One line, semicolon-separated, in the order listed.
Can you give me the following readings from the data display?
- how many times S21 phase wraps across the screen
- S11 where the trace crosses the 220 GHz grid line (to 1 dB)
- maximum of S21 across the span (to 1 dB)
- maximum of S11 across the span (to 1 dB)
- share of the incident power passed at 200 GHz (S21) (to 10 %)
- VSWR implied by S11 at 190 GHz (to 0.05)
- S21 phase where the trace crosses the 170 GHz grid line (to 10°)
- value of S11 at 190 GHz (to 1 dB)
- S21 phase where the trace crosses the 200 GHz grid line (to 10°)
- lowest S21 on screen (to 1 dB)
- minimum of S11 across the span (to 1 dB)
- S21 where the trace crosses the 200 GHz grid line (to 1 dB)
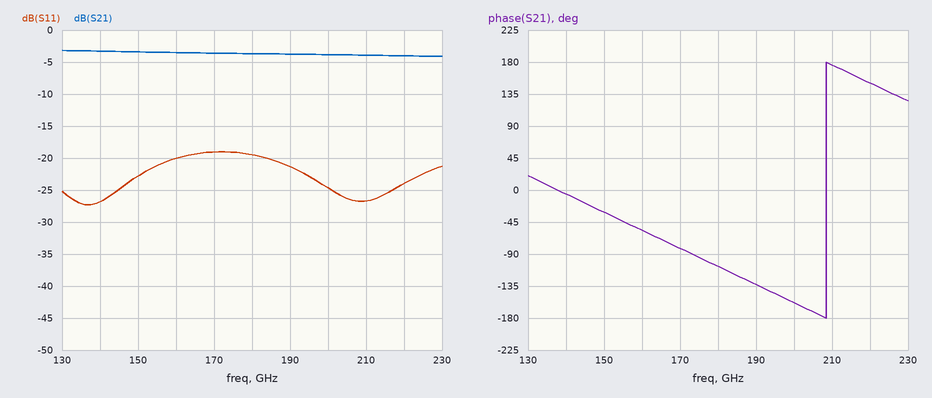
1; -24 dB; -3 dB; -19 dB; 40 %; 1.20; -80°; -21 dB; -160°; -4 dB; -27 dB; -4 dB
